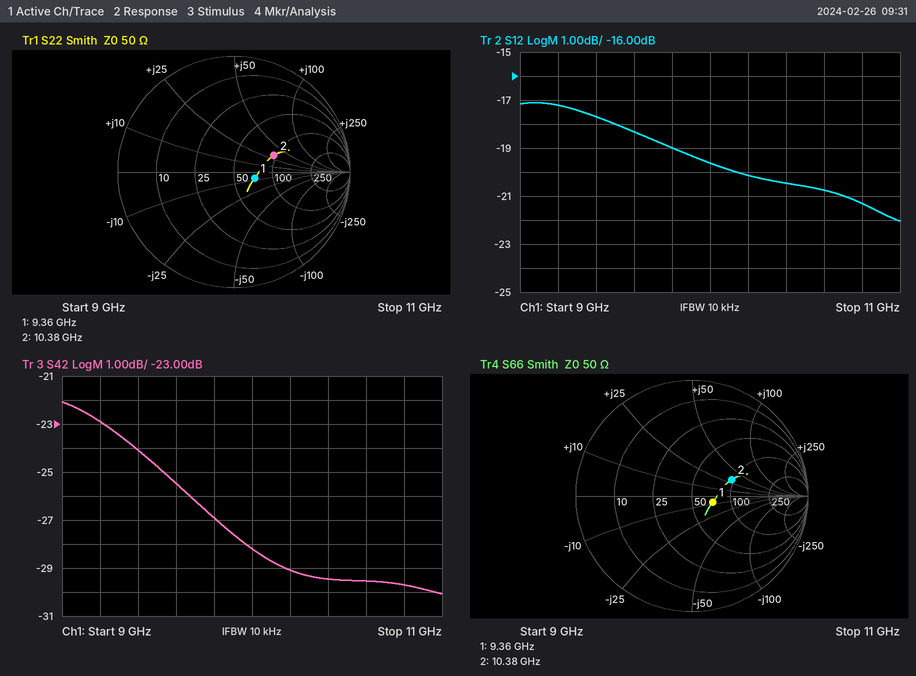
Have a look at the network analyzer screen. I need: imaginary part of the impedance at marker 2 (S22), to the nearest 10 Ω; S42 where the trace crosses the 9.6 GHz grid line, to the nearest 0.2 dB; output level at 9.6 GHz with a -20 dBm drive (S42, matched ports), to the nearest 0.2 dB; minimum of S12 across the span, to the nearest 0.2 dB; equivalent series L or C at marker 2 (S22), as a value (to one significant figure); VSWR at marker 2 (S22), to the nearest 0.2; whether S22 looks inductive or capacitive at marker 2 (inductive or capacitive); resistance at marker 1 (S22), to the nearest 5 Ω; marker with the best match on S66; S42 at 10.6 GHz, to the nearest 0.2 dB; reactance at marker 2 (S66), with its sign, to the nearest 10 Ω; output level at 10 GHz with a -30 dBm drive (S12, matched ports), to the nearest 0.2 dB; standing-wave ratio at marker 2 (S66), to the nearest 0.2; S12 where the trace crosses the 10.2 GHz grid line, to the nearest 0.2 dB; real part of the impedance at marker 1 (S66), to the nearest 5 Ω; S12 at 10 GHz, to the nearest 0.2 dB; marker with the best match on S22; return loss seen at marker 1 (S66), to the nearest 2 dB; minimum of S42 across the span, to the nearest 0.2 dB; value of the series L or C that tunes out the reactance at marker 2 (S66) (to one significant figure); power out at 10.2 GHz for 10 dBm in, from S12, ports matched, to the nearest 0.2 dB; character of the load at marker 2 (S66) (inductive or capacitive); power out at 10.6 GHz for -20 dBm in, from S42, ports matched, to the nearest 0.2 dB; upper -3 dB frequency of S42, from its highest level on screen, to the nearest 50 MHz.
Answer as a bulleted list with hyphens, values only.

- +30 Ω
- -25.4 dB
- -45.4 dBm
- -22.0 dB
- 500 pH
- 2.2
- inductive
- 70 Ω
- marker 1
- -29.6 dB
- +30 Ω
- -49.6 dBm
- 2.2
- -20.2 dB
- 70 Ω
- -19.6 dB
- marker 1
- 14 dB
- -30.0 dB
- 500 fF
- -10.2 dBm
- inductive
- -49.6 dBm
- 9.55 GHz
